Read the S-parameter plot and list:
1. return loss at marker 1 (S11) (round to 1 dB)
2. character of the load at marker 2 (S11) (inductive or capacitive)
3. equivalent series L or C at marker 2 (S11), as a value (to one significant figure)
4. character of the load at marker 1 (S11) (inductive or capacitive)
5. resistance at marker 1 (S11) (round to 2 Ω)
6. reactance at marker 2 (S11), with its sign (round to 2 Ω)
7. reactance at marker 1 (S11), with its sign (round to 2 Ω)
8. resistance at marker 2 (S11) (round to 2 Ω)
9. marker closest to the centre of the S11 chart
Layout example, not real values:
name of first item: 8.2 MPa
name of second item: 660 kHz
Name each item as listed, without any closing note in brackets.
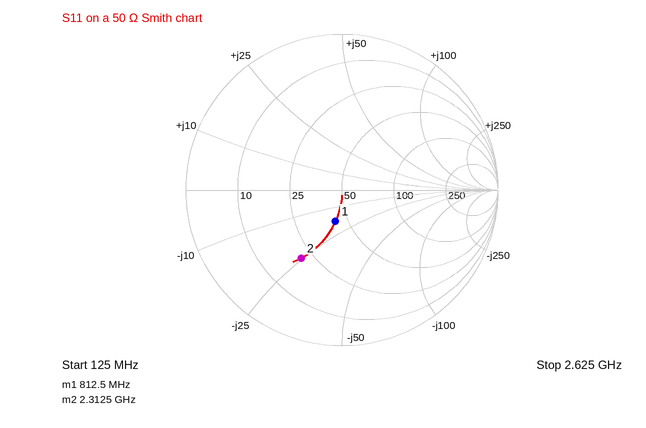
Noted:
return loss at marker 1 (S11): 14 dB
character of the load at marker 2 (S11): capacitive
equivalent series L or C at marker 2 (S11), as a value: 3 pF
character of the load at marker 1 (S11): capacitive
resistance at marker 1 (S11): 42 Ω
reactance at marker 2 (S11), with its sign: -24 Ω
reactance at marker 1 (S11), with its sign: -18 Ω
resistance at marker 2 (S11): 20 Ω
marker closest to the centre of the S11 chart: marker 1
